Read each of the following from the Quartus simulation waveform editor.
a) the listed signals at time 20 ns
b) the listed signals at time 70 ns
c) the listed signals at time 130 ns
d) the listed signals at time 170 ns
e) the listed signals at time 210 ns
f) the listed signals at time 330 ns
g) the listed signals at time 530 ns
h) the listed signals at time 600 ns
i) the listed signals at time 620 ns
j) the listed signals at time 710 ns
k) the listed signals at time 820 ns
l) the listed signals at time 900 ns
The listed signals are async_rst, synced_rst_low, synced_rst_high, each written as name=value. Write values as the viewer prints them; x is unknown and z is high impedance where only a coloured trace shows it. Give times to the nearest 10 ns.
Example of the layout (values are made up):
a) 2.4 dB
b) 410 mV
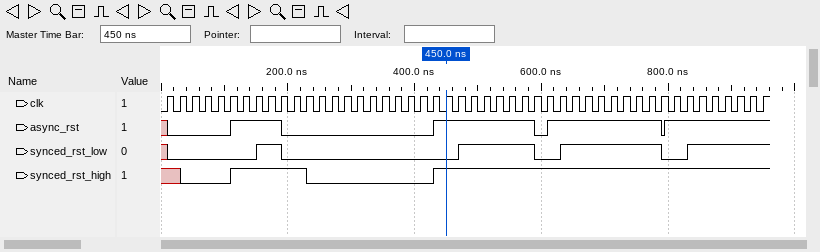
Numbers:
a) async_rst=0, synced_rst_low=0, synced_rst_high=x
b) async_rst=0, synced_rst_low=0, synced_rst_high=0
c) async_rst=1, synced_rst_low=0, synced_rst_high=1
d) async_rst=1, synced_rst_low=1, synced_rst_high=1
e) async_rst=0, synced_rst_low=0, synced_rst_high=1
f) async_rst=0, synced_rst_low=0, synced_rst_high=0
g) async_rst=1, synced_rst_low=1, synced_rst_high=1
h) async_rst=0, synced_rst_low=0, synced_rst_high=1
i) async_rst=1, synced_rst_low=0, synced_rst_high=1
j) async_rst=1, synced_rst_low=1, synced_rst_high=1
k) async_rst=1, synced_rst_low=0, synced_rst_high=1
l) async_rst=1, synced_rst_low=1, synced_rst_high=1
